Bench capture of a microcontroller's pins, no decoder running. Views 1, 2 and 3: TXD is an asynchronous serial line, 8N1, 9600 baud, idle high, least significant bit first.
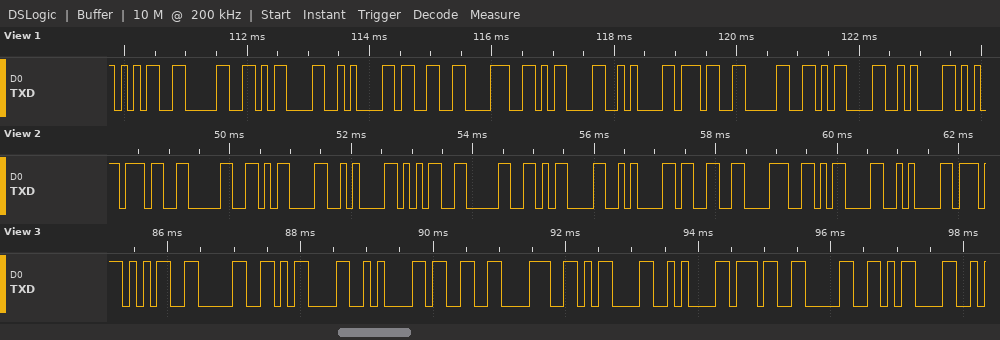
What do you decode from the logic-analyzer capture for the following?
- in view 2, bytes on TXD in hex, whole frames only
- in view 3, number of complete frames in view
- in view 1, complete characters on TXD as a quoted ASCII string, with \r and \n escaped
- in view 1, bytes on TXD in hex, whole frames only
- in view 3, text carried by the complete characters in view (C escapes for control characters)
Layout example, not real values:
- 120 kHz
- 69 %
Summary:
- 0x37 0x30 0x0D 0x0A 0x35 0x30 0x0D 0x0A 0x33 0x38 0x0D 0x0A
- 11
- "50\r\n38\r\n70\r\n"
- 35 30 0D 0A 33 38 0D 0A 37 30 0D 0A
- "50\r\n38\r\n70\r"
